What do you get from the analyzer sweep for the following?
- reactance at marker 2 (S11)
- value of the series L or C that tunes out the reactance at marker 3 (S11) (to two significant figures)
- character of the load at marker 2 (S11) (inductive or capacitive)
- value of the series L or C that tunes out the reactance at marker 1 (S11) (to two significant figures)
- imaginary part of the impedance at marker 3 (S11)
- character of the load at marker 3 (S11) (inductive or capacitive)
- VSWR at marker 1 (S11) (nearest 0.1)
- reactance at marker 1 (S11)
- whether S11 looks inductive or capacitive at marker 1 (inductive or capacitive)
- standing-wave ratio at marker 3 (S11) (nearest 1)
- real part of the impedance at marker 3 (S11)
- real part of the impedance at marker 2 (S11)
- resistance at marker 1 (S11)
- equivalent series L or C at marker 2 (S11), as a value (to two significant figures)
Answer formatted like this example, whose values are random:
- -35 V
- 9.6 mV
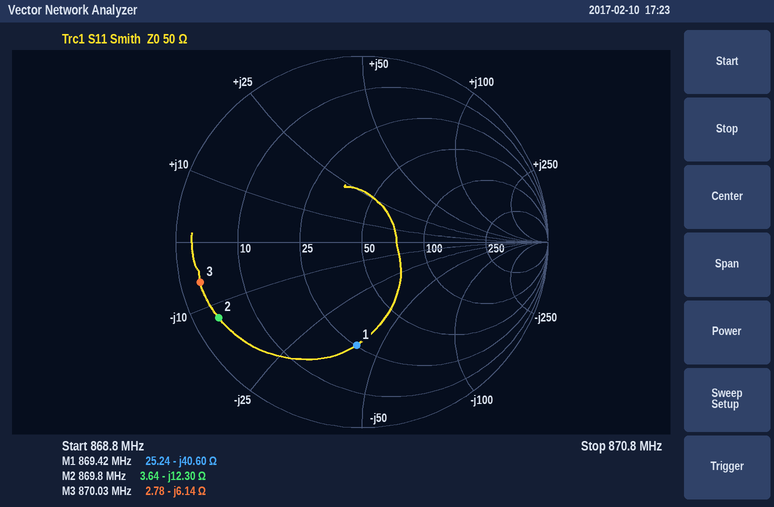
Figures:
- -12.30 Ω
- 1.1 nH
- capacitive
- 7.4 nH
- -6.14 Ω
- capacitive
- 3.5
- -40.60 Ω
- capacitive
- 18
- 2.78 Ω
- 3.64 Ω
- 25.24 Ω
- 15 pF
